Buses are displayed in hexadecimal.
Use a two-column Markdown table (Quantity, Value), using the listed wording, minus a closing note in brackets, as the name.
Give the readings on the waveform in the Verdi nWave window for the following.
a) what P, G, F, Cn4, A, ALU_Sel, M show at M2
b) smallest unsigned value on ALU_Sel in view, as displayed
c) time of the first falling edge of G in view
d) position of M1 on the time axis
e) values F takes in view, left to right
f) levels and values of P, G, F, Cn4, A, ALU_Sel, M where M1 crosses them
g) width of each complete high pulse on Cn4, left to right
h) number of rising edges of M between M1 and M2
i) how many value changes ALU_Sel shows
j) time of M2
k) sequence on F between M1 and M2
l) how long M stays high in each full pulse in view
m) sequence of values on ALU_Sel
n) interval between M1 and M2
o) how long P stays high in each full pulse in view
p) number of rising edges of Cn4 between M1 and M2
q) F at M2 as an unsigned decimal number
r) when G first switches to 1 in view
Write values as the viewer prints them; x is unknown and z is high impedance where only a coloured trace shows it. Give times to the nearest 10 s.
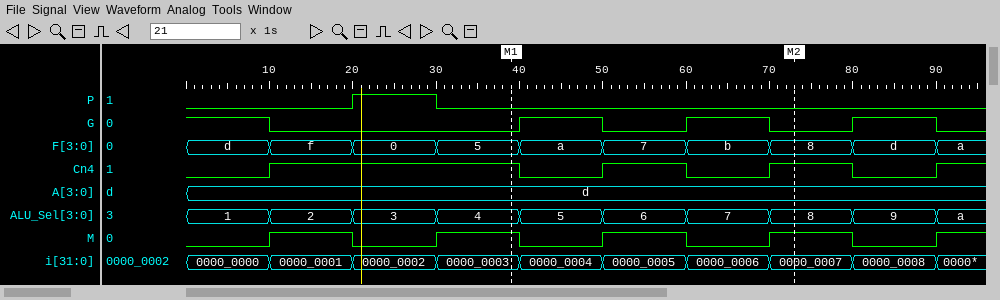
| Quantity | Value |
|---|---|
| what P, G, F, Cn4, A, ALU_Sel, M show at M2 | P=0, G=0, F=8, Cn4=1, A=d, ALU_Sel=8, M=1 |
| smallest unsigned value on ALU_Sel in view, as displayed | 1 |
| time of the first falling edge of G in view | 10 s |
| position of M1 on the time axis | 40 s |
| values F takes in view, left to right | d, f, 0, 5, a, 7, b, 8, d, a |
| levels and values of P, G, F, Cn4, A, ALU_Sel, M where M1 crosses them | P=0, G=0, F=5, Cn4=1, A=d, ALU_Sel=4, M=1 |
| width of each complete high pulse on Cn4, left to right | 30 s, 10 s, 10 s |
| number of rising edges of M between M1 and M2 | 2 |
| how many value changes ALU_Sel shows | 9 |
| time of M2 | 70 s |
| sequence on F between M1 and M2 | 5, a, 7, b, 8 |
| how long M stays high in each full pulse in view | 10 s, 10 s, 10 s, 10 s |
| sequence of values on ALU_Sel | 1, 2, 3, 4, 5, 6, 7, 8, 9, a |
| interval between M1 and M2 | 30 s |
| how long P stays high in each full pulse in view | 10 s |
| number of rising edges of Cn4 between M1 and M2 | 2 |
| F at M2 as an unsigned decimal number | 8 |
| when G first switches to 1 in view | 40 s |
